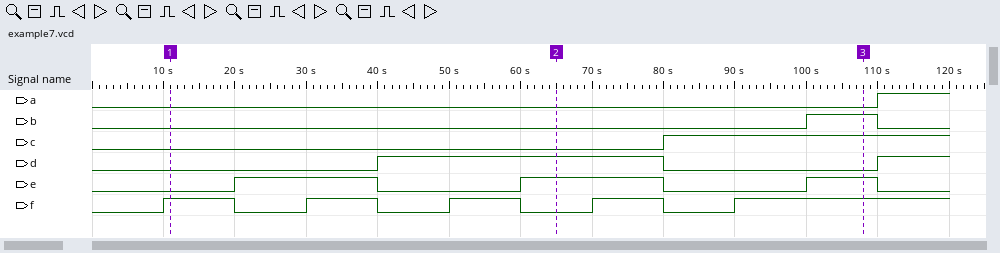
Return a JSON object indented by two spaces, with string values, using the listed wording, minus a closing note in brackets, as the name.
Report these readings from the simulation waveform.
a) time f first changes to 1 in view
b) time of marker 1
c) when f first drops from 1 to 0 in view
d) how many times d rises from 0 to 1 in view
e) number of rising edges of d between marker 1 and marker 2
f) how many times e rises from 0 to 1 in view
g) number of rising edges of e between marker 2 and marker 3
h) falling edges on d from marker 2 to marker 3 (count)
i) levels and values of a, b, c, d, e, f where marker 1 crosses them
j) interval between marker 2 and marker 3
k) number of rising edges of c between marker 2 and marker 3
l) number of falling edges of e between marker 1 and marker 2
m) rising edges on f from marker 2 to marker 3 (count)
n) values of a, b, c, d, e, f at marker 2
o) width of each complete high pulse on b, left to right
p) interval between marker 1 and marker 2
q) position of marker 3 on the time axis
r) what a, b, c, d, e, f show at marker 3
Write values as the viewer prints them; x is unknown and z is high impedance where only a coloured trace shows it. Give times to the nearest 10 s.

{
  "time f first changes to 1 in view": "10 s",
  "time of marker 1": "10 s",
  "when f first drops from 1 to 0 in view": "20 s",
  "how many times d rises from 0 to 1 in view": "2",
  "number of rising edges of d between marker 1 and marker 2": "1",
  "how many times e rises from 0 to 1 in view": "3",
  "number of rising edges of e between marker 2 and marker 3": "1",
  "falling edges on d from marker 2 to marker 3": "1",
  "levels and values of a, b, c, d, e, f where marker 1 crosses them": "a=0, b=0, c=0, d=0, e=0, f=1",
  "interval between marker 2 and marker 3": "40 s",
  "number of rising edges of c between marker 2 and marker 3": "1",
  "number of falling edges of e between marker 1 and marker 2": "1",
  "rising edges on f from marker 2 to marker 3": "2",
  "values of a, b, c, d, e, f at marker 2": "a=0, b=0, c=0, d=1, e=1, f=0",
  "width of each complete high pulse on b, left to right": "10 s",
  "interval between marker 1 and marker 2": "50 s",
  "position of marker 3 on the time axis": "110 s",
  "what a, b, c, d, e, f show at marker 3": "a=0, b=1, c=1, d=0, e=1, f=1"
}
